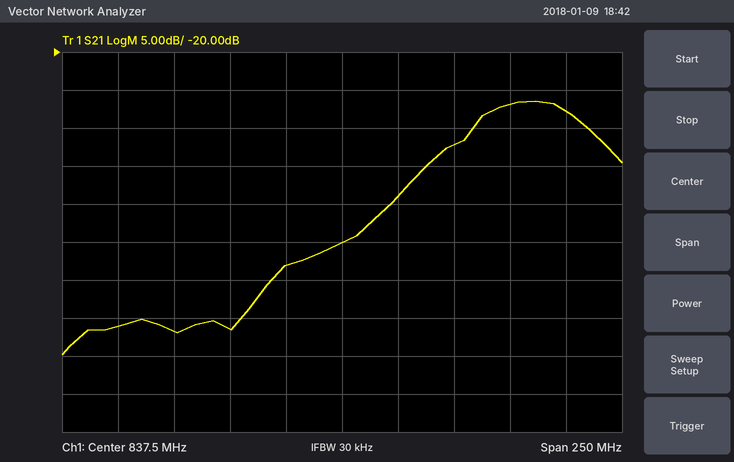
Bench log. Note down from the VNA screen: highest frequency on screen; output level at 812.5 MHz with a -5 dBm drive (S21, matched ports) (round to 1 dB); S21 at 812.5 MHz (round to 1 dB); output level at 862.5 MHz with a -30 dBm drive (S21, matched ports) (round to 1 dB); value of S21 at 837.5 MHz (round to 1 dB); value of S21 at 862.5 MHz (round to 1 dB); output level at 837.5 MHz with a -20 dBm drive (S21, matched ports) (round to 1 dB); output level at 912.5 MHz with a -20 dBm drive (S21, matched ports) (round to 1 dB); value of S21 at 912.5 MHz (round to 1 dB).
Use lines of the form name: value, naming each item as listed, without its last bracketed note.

highest frequency on screen: 962.5 MHz
output level at 812.5 MHz with a -5 dBm drive (S21, matched ports): -53 dBm
S21 at 812.5 MHz: -48 dB
output level at 862.5 MHz with a -30 dBm drive (S21, matched ports): -69 dBm
value of S21 at 837.5 MHz: -45 dB
value of S21 at 862.5 MHz: -39 dB
output level at 837.5 MHz with a -20 dBm drive (S21, matched ports): -65 dBm
output level at 912.5 MHz with a -20 dBm drive (S21, matched ports): -47 dBm
value of S21 at 912.5 MHz: -27 dB
